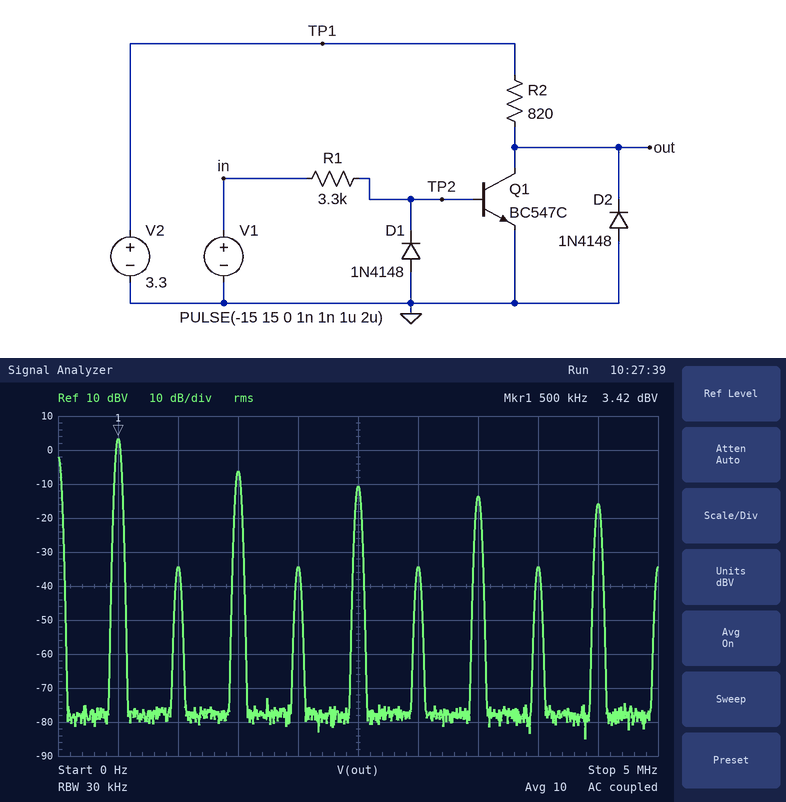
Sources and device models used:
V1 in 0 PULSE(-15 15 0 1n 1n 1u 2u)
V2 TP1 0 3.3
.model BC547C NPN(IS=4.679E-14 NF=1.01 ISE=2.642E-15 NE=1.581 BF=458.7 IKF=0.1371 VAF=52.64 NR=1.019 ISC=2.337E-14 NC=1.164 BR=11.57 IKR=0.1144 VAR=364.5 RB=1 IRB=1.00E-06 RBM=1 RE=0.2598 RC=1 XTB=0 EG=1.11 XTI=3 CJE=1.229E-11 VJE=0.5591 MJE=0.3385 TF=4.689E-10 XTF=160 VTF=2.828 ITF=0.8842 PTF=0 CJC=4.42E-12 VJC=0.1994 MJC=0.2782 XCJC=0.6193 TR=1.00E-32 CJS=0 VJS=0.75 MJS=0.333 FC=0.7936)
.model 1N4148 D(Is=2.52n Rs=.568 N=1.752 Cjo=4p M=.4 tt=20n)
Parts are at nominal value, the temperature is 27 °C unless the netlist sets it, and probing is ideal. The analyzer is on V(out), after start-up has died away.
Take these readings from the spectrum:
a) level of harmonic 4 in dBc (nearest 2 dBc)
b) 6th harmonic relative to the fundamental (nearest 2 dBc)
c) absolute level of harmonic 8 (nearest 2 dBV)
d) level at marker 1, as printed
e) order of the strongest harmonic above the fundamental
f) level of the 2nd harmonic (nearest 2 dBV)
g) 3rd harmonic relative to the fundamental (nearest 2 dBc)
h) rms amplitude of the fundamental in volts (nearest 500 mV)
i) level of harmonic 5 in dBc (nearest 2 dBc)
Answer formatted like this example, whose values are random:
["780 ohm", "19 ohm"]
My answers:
["-38 dBc", "-38 dBc", "-34 dBV", "3.42 dBV", "3", "-34 dBV", "-10 dBc", "1.5 V", "-14 dBc"]
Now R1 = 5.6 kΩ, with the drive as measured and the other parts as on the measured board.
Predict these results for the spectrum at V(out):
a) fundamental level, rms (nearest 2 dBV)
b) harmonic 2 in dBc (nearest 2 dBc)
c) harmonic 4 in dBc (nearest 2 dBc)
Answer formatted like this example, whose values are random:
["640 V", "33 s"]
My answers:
["4 dBV", "-34 dBc", "-34 dBc"]
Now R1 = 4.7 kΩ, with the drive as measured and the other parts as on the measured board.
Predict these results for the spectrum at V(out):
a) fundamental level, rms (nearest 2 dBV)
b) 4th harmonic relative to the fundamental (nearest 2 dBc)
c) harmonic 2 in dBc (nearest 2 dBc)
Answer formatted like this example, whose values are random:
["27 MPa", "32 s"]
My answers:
["4 dBV", "-36 dBc", "-36 dBc"]
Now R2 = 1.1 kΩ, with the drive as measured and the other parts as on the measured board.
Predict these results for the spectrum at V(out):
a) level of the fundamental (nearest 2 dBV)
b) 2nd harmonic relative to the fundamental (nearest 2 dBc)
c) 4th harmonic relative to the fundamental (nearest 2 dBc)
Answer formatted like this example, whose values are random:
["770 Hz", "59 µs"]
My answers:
["4 dBV", "-40 dBc", "-40 dBc"]
